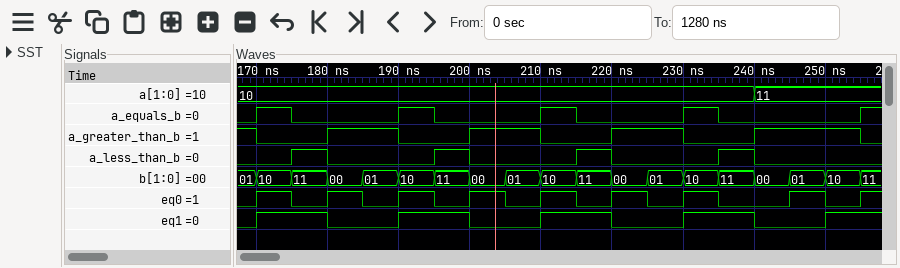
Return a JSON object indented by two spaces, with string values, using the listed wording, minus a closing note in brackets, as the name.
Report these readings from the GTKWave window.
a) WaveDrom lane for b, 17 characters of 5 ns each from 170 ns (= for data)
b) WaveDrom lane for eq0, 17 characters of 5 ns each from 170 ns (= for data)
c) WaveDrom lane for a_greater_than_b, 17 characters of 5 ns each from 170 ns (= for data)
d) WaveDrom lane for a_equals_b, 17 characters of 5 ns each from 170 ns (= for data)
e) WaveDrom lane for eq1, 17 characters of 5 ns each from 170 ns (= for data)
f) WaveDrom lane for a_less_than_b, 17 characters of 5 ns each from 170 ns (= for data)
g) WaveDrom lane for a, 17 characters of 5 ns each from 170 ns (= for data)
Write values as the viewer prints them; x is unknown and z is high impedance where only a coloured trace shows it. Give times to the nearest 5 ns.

{
  "WaveDrom lane for b, 17 characters of 5 ns each from 170 ns": "{name: 'b', wave: '=================', data: '10 11 00 01 10 11 00 01 10 11 00 01 10 11 00 01 10'}",
  "WaveDrom lane for eq0, 17 characters of 5 ns each from 170 ns": "{name: 'eq0', wave: '10101010101010.10'}",
  "WaveDrom lane for a_greater_than_b, 17 characters of 5 ns each from 170 ns": "{name: 'a_greater_than_b', wave: '0.1.0.1.0.1.0.1..'}",
  "WaveDrom lane for a_equals_b, 17 characters of 5 ns each from 170 ns": "{name: 'a_equals_b', wave: '10..10..10..10...'}",
  "WaveDrom lane for eq1, 17 characters of 5 ns each from 170 ns": "{name: 'eq1', wave: '1.0.1.0.1.0.1.0.1'}",
  "WaveDrom lane for a_less_than_b, 17 characters of 5 ns each from 170 ns": "{name: 'a_less_than_b', wave: '010..10..10..10..'}",
  "WaveDrom lane for a, 17 characters of 5 ns each from 170 ns": "{name: 'a', wave: '=.............=..', data: '10 11'}"
}
